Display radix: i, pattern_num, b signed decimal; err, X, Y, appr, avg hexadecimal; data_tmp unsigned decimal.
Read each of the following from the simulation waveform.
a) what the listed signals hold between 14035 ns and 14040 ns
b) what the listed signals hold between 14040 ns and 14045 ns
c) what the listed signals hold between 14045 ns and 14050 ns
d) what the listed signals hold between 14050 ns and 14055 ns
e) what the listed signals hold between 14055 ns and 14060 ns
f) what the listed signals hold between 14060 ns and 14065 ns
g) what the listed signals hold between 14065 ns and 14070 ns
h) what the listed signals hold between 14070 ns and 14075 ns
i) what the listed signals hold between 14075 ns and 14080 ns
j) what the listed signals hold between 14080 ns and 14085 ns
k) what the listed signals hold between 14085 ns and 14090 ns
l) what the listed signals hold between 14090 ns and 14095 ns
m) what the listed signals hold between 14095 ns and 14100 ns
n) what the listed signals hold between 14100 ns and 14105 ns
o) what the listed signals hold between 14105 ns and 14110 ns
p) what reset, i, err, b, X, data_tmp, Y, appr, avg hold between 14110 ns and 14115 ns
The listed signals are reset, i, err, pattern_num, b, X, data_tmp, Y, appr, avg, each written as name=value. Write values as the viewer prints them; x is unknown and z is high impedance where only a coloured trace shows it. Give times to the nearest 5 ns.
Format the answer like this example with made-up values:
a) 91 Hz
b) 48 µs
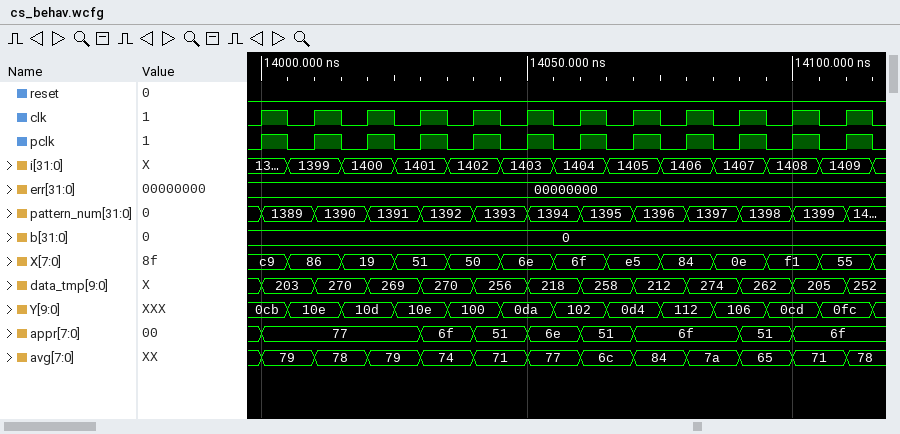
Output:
a) reset=0, i=1402, err=00000000, pattern_num=1392, b=0, X=50, data_tmp=270, Y=100, appr=6f, avg=74
b) reset=0, i=1402, err=00000000, pattern_num=1393, b=0, X=50, data_tmp=256, Y=100, appr=51, avg=71
c) reset=0, i=1403, err=00000000, pattern_num=1393, b=0, X=6e, data_tmp=256, Y=0da, appr=51, avg=71
d) reset=0, i=1403, err=00000000, pattern_num=1394, b=0, X=6e, data_tmp=218, Y=0da, appr=6e, avg=77
e) reset=0, i=1404, err=00000000, pattern_num=1394, b=0, X=6f, data_tmp=218, Y=102, appr=6e, avg=77
f) reset=0, i=1404, err=00000000, pattern_num=1395, b=0, X=6f, data_tmp=258, Y=102, appr=51, avg=6c
g) reset=0, i=1405, err=00000000, pattern_num=1395, b=0, X=e5, data_tmp=258, Y=0d4, appr=51, avg=6c
h) reset=0, i=1405, err=00000000, pattern_num=1396, b=0, X=e5, data_tmp=212, Y=0d4, appr=6f, avg=84
i) reset=0, i=1406, err=00000000, pattern_num=1396, b=0, X=84, data_tmp=212, Y=112, appr=6f, avg=84
j) reset=0, i=1406, err=00000000, pattern_num=1397, b=0, X=84, data_tmp=274, Y=112, appr=6f, avg=7a
k) reset=0, i=1407, err=00000000, pattern_num=1397, b=0, X=0e, data_tmp=274, Y=106, appr=6f, avg=7a
l) reset=0, i=1407, err=00000000, pattern_num=1398, b=0, X=0e, data_tmp=262, Y=106, appr=51, avg=65
m) reset=0, i=1408, err=00000000, pattern_num=1398, b=0, X=f1, data_tmp=262, Y=0cd, appr=51, avg=65
n) reset=0, i=1408, err=00000000, pattern_num=1399, b=0, X=f1, data_tmp=205, Y=0cd, appr=6f, avg=71
o) reset=0, i=1409, err=00000000, pattern_num=1399, b=0, X=55, data_tmp=205, Y=0fc, appr=6f, avg=71
p) reset=0, i=1409, err=00000000, b=0, X=55, data_tmp=252, Y=0fc, appr=6f, avg=78
